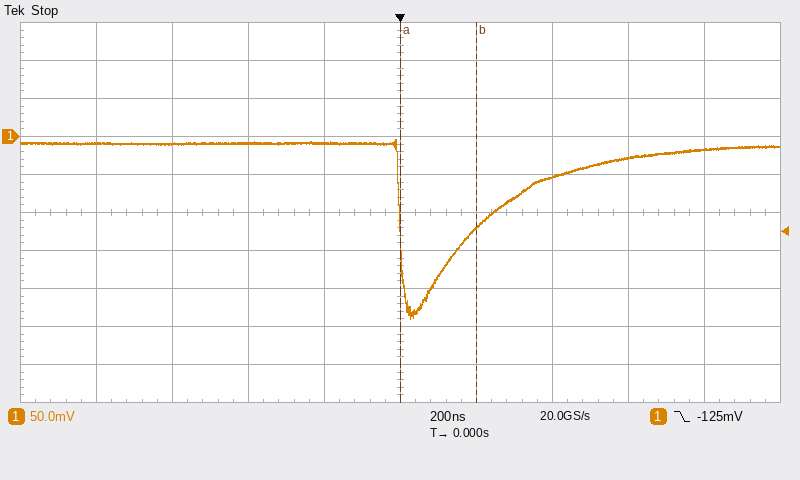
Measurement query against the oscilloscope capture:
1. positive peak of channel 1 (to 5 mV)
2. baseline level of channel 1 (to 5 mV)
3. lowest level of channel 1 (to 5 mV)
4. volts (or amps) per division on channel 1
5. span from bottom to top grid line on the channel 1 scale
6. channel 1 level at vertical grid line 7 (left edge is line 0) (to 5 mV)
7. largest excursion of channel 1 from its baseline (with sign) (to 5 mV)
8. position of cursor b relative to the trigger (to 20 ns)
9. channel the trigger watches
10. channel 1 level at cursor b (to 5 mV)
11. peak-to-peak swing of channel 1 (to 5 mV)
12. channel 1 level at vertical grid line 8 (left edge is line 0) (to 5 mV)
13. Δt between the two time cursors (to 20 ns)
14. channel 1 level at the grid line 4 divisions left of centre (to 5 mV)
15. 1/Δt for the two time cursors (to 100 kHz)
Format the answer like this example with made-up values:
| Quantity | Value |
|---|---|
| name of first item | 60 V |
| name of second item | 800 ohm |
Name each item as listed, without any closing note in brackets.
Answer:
| Quantity | Value |
|---|---|
| positive peak of channel 1 | -5 mV |
| baseline level of channel 1 | -10 mV |
| lowest level of channel 1 | -240 mV |
| volts (or amps) per division on channel 1 | 50 mV |
| span from bottom to top grid line on the channel 1 scale | 500 mV |
| channel 1 level at vertical grid line 7 (left edge is line 0) | -55 mV |
| largest excursion of channel 1 from its baseline (with sign) | -230 mV |
| position of cursor b relative to the trigger | +200 ns |
| channel the trigger watches | channel 1 |
| channel 1 level at cursor b | -120 mV |
| peak-to-peak swing of channel 1 | 235 mV |
| channel 1 level at vertical grid line 8 (left edge is line 0) | -30 mV |
| Δt between the two time cursors | 200 ns |
| channel 1 level at the grid line 4 divisions left of centre | -10 mV |
| 1/Δt for the two time cursors | 5.0 MHz |
